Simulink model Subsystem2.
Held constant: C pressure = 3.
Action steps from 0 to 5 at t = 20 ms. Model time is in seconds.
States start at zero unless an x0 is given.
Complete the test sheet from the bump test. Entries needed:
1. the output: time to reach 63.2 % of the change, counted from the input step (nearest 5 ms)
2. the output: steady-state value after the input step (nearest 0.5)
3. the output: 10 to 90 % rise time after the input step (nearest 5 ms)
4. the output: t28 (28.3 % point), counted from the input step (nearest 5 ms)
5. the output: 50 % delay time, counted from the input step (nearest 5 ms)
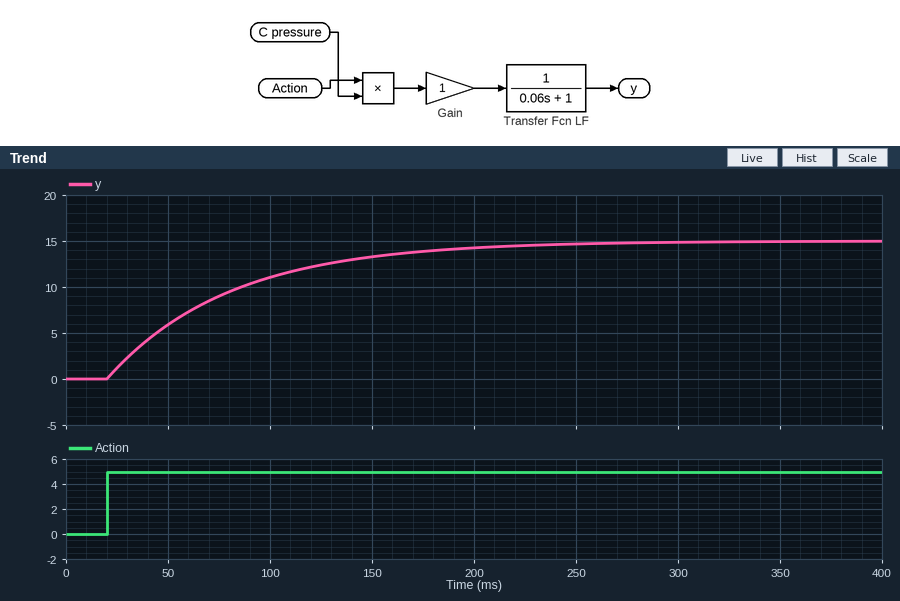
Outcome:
60 ms
15.0
130 ms
20 ms
40 ms
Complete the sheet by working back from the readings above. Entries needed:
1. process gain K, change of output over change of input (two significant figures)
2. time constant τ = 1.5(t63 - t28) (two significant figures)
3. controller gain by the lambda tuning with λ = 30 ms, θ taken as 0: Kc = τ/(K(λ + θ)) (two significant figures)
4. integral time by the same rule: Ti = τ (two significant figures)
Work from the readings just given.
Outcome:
3.0
60 ms
0.67
60 ms
